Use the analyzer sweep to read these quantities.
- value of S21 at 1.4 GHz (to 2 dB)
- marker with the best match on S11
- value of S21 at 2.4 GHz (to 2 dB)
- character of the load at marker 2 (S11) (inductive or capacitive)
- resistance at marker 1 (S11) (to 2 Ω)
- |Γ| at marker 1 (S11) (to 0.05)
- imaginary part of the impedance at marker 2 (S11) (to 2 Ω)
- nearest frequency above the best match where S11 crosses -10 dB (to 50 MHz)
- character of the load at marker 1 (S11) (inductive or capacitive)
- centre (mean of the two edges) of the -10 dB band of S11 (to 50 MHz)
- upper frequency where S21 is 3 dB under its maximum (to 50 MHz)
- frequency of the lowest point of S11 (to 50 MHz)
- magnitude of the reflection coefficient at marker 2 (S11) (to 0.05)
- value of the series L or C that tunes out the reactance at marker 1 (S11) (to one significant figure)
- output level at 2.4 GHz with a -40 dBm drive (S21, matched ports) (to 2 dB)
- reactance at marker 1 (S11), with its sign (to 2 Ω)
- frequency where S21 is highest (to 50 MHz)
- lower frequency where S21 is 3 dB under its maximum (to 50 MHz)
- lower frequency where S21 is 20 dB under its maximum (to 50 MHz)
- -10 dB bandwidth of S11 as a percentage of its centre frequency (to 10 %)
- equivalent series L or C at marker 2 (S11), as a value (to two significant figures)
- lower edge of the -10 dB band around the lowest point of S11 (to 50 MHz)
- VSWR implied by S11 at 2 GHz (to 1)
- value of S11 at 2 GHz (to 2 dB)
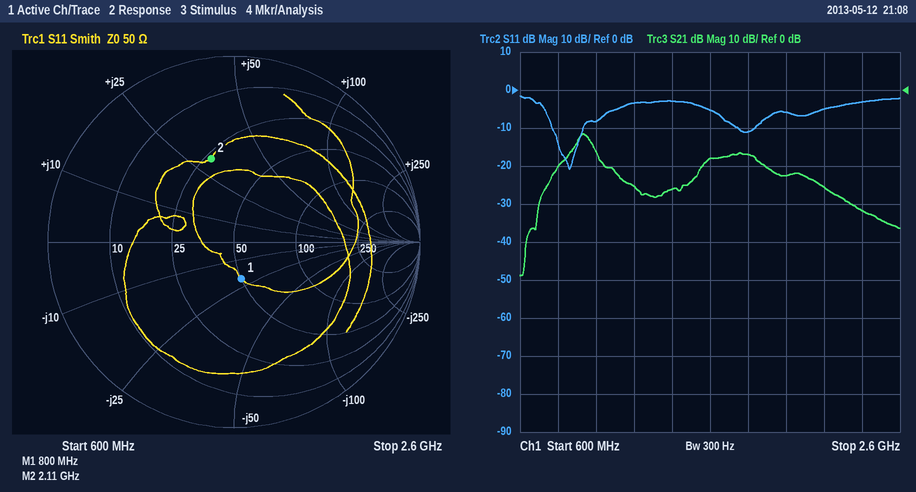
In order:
-26 dB
marker 1
-32 dB
inductive
50 Ω
0.20
+30 Ω
950 MHz
capacitive
850 MHz
1.00 GHz
850 MHz
0.45
4 nH
-72 dBm
-20 Ω
950 MHz
900 MHz
700 MHz
20 %
2.3 nH
750 MHz
3
-6 dB
